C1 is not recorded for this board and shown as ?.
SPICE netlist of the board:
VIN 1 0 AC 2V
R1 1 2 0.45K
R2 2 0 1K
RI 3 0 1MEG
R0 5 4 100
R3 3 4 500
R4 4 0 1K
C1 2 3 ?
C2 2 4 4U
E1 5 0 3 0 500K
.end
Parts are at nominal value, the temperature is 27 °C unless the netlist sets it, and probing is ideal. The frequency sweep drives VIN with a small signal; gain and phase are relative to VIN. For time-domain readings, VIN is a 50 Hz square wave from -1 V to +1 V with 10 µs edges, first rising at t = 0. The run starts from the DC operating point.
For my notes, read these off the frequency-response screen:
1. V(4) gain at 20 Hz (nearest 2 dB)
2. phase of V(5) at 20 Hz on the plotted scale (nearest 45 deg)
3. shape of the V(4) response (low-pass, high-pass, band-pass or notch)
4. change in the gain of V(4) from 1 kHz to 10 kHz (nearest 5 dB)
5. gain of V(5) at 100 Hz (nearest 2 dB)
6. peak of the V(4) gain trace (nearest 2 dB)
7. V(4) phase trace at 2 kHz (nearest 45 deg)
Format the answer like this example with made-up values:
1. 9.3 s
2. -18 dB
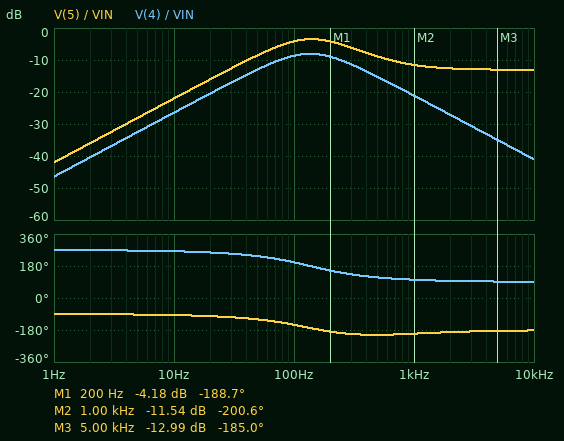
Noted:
1. -20 dB
2. -90 deg
3. band-pass
4. -20 dB
5. -4 dB
6. -8 dB
7. 90 deg
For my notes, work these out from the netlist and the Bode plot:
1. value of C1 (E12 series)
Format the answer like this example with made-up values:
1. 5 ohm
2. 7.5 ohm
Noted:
1. 2.2 µF
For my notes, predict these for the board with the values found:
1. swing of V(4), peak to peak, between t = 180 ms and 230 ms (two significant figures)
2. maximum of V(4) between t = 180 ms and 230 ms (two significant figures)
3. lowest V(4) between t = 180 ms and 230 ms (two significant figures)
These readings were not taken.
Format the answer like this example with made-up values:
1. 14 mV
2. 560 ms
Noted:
1. 1.1 V
2. 540 mV
3. -540 mV
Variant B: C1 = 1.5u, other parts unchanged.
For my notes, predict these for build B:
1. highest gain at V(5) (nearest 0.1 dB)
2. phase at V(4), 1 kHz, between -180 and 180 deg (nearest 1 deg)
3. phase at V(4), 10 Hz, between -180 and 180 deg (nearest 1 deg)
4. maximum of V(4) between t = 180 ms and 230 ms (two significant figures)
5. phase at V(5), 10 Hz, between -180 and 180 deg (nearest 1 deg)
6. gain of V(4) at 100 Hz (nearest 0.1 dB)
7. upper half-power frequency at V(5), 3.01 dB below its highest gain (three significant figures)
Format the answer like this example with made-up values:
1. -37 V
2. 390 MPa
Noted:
1. -4.9 dB
2. 107 deg
3. -96 deg
4. 430 mV
5. -95 deg
6. -11.7 dB
7. 427 Hz
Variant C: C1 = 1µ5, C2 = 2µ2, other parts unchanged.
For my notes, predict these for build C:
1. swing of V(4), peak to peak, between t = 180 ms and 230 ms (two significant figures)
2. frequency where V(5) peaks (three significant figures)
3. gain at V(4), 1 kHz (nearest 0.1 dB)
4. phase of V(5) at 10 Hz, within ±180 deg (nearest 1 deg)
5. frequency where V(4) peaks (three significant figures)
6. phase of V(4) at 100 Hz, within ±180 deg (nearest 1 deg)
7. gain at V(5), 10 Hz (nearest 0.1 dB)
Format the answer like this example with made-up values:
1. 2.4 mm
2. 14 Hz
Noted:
1. 1.2 V
2. 228 Hz
3. -16.0 dB
4. -94 deg
5. 222 Hz
6. -132 deg
7. -25.7 dB
